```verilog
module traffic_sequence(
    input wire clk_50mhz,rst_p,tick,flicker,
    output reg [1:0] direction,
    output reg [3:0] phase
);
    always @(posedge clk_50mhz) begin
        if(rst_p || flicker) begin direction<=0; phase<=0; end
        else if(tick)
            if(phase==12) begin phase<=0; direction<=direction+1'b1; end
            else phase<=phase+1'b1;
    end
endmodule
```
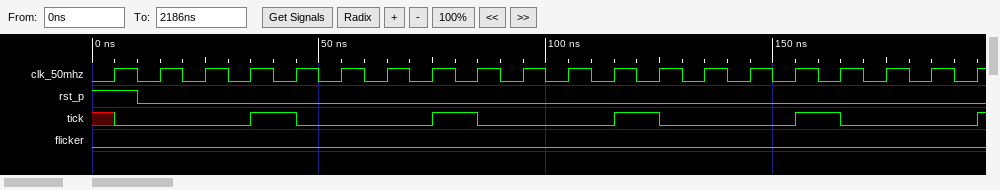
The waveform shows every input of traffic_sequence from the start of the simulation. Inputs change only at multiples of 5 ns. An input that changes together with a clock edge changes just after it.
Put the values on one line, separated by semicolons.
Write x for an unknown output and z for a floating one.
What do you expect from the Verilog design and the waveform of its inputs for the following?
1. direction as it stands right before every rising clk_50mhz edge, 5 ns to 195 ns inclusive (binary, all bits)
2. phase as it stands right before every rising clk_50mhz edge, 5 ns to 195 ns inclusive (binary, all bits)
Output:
x, 00, 00, 00, 00, 00, 00, 00, 00, 00, 00, 00, 00, 00, 00, 00, 00, 00, 00, 00; x, 0000, 0000, 0000, 0000, 0001, 0001, 0001, 0001, 0010, 0010, 0010, 0010, 0011, 0011, 0011, 0011, 0100, 0100, 0100
